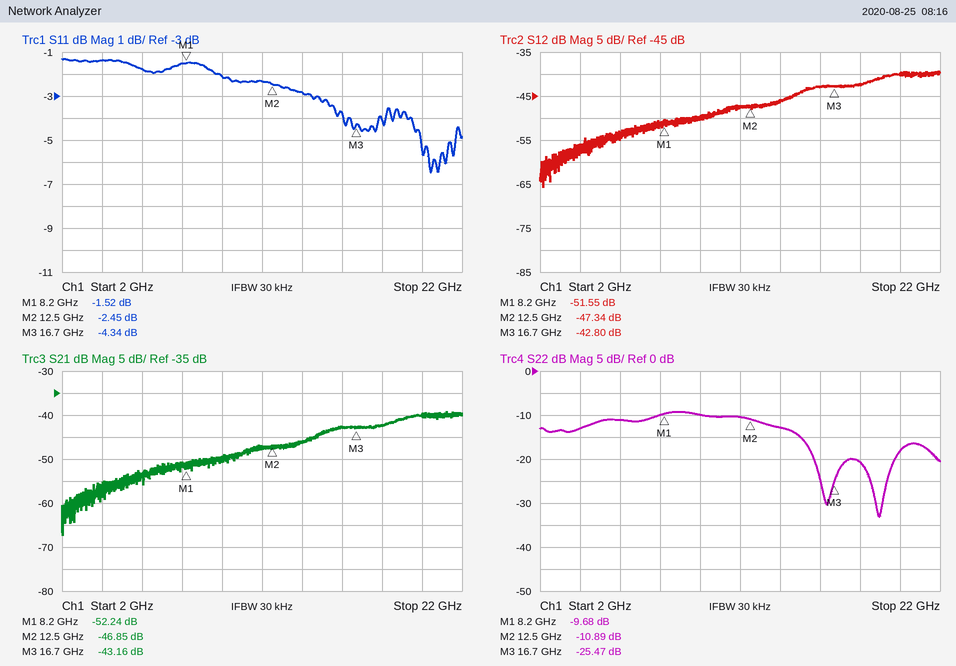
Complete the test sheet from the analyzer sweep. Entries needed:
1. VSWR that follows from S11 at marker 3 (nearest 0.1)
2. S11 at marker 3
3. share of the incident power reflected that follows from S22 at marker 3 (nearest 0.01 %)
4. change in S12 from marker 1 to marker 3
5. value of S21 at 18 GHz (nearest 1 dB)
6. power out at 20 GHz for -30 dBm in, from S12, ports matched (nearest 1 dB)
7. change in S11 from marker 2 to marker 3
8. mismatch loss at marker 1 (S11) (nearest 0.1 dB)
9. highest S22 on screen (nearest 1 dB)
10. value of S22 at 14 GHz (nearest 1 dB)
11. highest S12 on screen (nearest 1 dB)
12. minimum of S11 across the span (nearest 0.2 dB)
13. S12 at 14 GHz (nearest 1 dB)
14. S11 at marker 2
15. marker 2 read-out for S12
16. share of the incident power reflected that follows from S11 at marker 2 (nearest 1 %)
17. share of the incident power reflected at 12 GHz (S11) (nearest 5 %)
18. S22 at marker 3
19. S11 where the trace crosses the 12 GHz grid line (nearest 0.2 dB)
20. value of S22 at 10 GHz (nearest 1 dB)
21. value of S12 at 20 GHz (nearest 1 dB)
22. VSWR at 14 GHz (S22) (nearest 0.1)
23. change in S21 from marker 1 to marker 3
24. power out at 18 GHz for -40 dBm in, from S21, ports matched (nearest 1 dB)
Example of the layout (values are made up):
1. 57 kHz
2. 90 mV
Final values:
1. 4.1
2. -4.34 dB
3. 0.28 %
4. 8.75 dB
5. -42 dB
6. -70 dBm
7. -1.89 dB
8. 5.3 dB
9. -9 dB
10. -13 dB
11. -39 dB
12. -6.4 dB
13. -46 dB
14. -2.45 dB
15. -47.34 dB
16. 57 %
17. 60 %
18. -25.47 dB
19. -2.4 dB
20. -10 dB
21. -40 dB
22. 1.6
23. 9.08 dB
24. -82 dBm
